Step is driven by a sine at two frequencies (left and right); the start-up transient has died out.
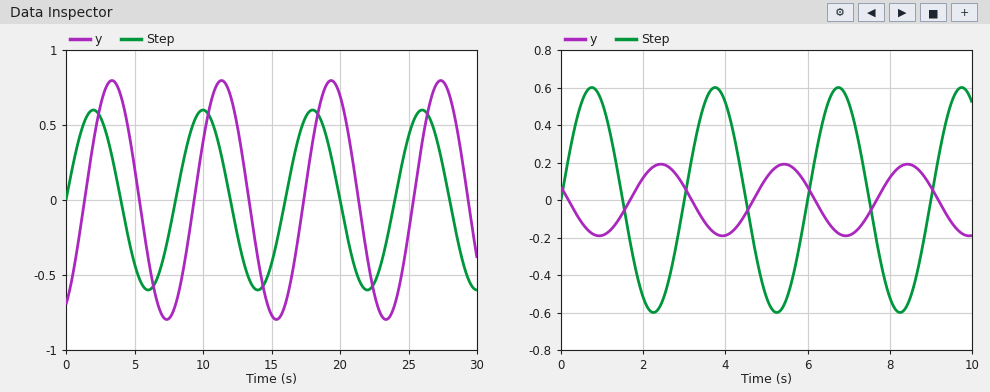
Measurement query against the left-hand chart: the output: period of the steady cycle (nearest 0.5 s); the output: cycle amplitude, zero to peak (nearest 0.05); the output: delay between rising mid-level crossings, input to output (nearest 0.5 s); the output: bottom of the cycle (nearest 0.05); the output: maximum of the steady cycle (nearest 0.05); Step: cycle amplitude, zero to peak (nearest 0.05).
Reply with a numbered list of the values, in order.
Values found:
1. 8.0 s
2. 0.80
3. 1.5 s
4. -0.80
5. 0.80
6. 0.60
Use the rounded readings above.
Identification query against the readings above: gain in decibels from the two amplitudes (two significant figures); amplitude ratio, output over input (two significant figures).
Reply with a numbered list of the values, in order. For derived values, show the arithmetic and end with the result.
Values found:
1. 20 log10(0.8 / 0.6) = 2.5 dB
2. 0.8 / 0.6 = 1.3
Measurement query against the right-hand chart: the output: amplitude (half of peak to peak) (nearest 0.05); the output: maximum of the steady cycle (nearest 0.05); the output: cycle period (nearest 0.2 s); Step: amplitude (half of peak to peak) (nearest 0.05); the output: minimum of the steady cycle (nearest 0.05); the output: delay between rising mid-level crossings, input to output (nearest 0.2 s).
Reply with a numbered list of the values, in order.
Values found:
1. 0.20
2. 0.20
3. 3.0 s
4. 0.60
5. -0.20
6. 1.6 s
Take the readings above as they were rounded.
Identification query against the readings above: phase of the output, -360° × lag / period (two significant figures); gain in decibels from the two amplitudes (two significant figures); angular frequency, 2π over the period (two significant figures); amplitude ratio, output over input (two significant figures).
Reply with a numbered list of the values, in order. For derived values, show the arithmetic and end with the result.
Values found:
1. -360 × 1.6 / 3 = -190°
2. 20 log10(0.2 / 0.6) = -9.5 dB
3. 2π / 3 = 2.1 rad/s
4. 0.2 / 0.6 = 0.33
